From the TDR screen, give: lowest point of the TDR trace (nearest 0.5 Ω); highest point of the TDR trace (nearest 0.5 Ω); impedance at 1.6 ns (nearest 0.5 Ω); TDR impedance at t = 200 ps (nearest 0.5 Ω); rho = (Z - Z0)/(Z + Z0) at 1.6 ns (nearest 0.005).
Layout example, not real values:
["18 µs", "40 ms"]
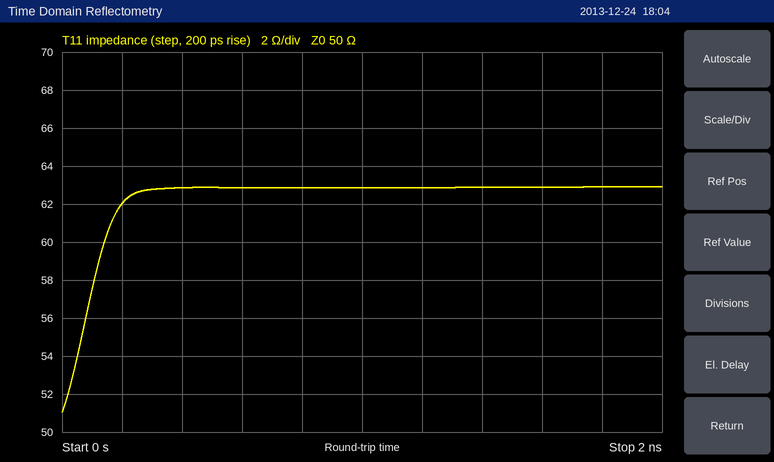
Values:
["51.0 Ω", "63.0 Ω", "63.0 Ω", "62.0 Ω", "+0.115"]
